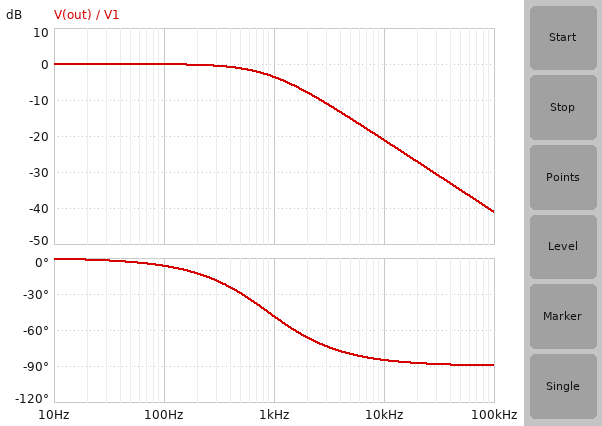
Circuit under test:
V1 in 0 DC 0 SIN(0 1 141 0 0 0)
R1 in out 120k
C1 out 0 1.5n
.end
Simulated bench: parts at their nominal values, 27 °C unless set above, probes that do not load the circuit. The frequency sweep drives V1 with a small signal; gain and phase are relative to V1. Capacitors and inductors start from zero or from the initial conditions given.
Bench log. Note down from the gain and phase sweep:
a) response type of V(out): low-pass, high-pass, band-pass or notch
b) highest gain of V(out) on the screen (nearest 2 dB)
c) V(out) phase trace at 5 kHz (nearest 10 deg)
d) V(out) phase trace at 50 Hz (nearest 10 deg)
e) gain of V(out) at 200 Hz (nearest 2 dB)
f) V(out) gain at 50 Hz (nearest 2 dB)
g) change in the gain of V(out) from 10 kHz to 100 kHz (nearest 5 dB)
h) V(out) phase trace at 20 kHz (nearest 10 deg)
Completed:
low-pass
0 dB
-80 deg
0 deg
0 dB
0 dB
-20 dB
-90 deg
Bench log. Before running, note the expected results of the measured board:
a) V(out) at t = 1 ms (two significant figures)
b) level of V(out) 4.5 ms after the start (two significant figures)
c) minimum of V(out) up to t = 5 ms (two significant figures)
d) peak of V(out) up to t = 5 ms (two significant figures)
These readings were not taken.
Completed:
660 mV
-630 mV
-890 mV
990 mV
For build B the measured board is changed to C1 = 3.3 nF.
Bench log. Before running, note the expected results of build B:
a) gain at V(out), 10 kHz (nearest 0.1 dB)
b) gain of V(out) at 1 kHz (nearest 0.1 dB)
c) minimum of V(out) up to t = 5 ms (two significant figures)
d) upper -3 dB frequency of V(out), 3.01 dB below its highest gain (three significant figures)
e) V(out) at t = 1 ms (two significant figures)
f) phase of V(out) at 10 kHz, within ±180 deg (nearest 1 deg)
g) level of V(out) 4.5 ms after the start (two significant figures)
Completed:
-27.9 dB
-8.6 dB
-770 mV
402 Hz
520 mV
-88 deg
-460 mV
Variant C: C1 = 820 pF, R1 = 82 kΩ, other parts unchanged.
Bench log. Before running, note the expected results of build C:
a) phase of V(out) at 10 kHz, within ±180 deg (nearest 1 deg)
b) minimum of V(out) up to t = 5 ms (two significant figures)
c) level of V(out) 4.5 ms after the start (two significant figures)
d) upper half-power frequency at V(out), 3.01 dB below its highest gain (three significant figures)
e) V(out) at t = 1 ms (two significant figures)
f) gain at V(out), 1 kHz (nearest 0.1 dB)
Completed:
-77 deg
-940 mV
-710 mV
2.37 kHz
730 mV
-0.7 dB
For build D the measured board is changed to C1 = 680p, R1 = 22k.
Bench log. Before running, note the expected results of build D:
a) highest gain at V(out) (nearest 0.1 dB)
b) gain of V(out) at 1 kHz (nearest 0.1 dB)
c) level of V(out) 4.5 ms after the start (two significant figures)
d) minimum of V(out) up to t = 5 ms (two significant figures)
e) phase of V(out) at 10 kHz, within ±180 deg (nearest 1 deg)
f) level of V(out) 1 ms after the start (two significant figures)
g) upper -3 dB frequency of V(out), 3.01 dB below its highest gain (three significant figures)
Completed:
0 dB
0 dB
-740 mV
-960 mV
-43 deg
770 mV
10.6 kHz
